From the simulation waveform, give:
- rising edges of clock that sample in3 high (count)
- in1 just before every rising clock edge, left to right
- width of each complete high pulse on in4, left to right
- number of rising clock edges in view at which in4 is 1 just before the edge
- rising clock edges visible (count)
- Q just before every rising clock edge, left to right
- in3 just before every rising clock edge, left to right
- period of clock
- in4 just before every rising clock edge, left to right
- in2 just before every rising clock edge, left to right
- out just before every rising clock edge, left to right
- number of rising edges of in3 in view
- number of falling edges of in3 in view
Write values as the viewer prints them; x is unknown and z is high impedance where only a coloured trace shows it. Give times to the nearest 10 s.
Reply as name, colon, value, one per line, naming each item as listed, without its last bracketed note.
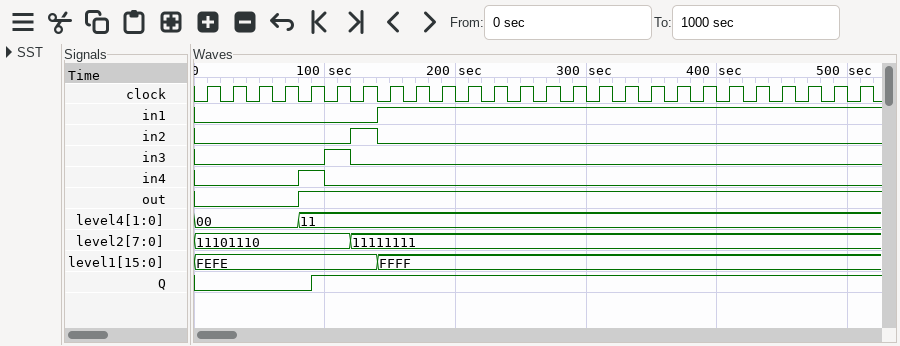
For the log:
rising edges of clock that sample in3 high: 1
in1 just before every rising clock edge, left to right: 0 0 0 0 0 0 0 1 1 1 1 1 1 1 1 1 1 1 1 1 1 1 1 1 1 1
width of each complete high pulse on in4, left to right: 20 s
number of rising clock edges in view at which in4 is 1 just before the edge: 1
rising clock edges visible: 26
Q just before every rising clock edge, left to right: 0 0 0 0 0 1 1 1 1 1 1 1 1 1 1 1 1 1 1 1 1 1 1 1 1 1
in3 just before every rising clock edge, left to right: 0 0 0 0 0 1 0 0 0 0 0 0 0 0 0 0 0 0 0 0 0 0 0 0 0 0
period of clock: 20 s
in4 just before every rising clock edge, left to right: 0 0 0 0 1 0 0 0 0 0 0 0 0 0 0 0 0 0 0 0 0 0 0 0 0 0
in2 just before every rising clock edge, left to right: 0 0 0 0 0 0 1 0 0 0 0 0 0 0 0 0 0 0 0 0 0 0 0 0 0 0
out just before every rising clock edge, left to right: 0 0 0 0 1 1 1 1 1 1 1 1 1 1 1 1 1 1 1 1 1 1 1 1 1 1
number of rising edges of in3 in view: 1
number of falling edges of in3 in view: 1
